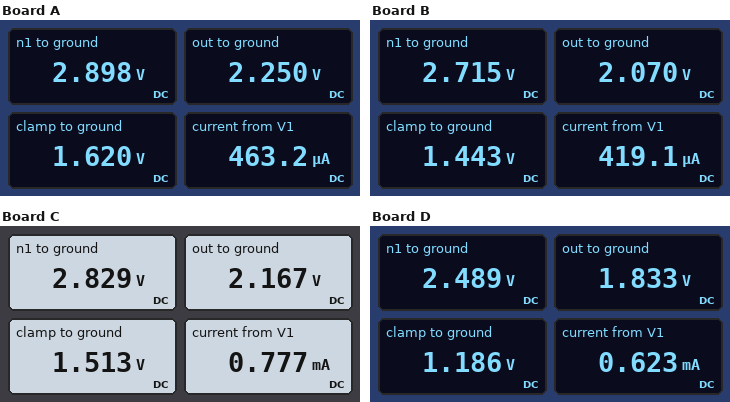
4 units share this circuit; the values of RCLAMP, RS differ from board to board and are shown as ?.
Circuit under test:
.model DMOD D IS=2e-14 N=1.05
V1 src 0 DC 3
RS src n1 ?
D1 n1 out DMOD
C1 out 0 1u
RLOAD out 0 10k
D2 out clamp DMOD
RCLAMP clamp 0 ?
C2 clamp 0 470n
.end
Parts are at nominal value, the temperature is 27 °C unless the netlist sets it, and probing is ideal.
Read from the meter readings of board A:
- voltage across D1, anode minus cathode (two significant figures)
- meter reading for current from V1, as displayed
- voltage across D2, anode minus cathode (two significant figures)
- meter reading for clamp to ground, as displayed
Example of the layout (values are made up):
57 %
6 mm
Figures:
650 mV
463.2 µA
630 mV
1.620 V
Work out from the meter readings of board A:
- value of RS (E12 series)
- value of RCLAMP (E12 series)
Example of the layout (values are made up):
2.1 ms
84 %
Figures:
220 Ω
6.8 kΩ
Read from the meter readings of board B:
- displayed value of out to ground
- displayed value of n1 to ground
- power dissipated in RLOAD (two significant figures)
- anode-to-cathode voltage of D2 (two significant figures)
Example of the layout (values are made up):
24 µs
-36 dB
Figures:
2.070 V
2.715 V
430 µW
630 mV
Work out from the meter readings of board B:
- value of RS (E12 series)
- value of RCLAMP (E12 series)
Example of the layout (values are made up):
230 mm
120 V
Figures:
680 Ω
6.8 kΩ
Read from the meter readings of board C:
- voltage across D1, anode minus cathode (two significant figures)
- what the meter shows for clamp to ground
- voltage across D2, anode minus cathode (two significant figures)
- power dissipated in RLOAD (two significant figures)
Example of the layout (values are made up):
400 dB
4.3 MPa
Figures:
660 mV
1.513 V
650 mV
470 µW
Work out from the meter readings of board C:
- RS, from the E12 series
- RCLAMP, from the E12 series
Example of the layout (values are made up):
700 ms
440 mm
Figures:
220 Ω
2.7 kΩ
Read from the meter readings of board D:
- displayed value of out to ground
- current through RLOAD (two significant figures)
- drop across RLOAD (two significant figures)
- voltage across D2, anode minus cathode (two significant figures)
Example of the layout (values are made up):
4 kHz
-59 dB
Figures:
1.833 V
180 µA
1.8 V
650 mV
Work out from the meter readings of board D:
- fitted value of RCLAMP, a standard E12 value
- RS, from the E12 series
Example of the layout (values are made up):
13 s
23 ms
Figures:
2.7 kΩ
820 Ω
